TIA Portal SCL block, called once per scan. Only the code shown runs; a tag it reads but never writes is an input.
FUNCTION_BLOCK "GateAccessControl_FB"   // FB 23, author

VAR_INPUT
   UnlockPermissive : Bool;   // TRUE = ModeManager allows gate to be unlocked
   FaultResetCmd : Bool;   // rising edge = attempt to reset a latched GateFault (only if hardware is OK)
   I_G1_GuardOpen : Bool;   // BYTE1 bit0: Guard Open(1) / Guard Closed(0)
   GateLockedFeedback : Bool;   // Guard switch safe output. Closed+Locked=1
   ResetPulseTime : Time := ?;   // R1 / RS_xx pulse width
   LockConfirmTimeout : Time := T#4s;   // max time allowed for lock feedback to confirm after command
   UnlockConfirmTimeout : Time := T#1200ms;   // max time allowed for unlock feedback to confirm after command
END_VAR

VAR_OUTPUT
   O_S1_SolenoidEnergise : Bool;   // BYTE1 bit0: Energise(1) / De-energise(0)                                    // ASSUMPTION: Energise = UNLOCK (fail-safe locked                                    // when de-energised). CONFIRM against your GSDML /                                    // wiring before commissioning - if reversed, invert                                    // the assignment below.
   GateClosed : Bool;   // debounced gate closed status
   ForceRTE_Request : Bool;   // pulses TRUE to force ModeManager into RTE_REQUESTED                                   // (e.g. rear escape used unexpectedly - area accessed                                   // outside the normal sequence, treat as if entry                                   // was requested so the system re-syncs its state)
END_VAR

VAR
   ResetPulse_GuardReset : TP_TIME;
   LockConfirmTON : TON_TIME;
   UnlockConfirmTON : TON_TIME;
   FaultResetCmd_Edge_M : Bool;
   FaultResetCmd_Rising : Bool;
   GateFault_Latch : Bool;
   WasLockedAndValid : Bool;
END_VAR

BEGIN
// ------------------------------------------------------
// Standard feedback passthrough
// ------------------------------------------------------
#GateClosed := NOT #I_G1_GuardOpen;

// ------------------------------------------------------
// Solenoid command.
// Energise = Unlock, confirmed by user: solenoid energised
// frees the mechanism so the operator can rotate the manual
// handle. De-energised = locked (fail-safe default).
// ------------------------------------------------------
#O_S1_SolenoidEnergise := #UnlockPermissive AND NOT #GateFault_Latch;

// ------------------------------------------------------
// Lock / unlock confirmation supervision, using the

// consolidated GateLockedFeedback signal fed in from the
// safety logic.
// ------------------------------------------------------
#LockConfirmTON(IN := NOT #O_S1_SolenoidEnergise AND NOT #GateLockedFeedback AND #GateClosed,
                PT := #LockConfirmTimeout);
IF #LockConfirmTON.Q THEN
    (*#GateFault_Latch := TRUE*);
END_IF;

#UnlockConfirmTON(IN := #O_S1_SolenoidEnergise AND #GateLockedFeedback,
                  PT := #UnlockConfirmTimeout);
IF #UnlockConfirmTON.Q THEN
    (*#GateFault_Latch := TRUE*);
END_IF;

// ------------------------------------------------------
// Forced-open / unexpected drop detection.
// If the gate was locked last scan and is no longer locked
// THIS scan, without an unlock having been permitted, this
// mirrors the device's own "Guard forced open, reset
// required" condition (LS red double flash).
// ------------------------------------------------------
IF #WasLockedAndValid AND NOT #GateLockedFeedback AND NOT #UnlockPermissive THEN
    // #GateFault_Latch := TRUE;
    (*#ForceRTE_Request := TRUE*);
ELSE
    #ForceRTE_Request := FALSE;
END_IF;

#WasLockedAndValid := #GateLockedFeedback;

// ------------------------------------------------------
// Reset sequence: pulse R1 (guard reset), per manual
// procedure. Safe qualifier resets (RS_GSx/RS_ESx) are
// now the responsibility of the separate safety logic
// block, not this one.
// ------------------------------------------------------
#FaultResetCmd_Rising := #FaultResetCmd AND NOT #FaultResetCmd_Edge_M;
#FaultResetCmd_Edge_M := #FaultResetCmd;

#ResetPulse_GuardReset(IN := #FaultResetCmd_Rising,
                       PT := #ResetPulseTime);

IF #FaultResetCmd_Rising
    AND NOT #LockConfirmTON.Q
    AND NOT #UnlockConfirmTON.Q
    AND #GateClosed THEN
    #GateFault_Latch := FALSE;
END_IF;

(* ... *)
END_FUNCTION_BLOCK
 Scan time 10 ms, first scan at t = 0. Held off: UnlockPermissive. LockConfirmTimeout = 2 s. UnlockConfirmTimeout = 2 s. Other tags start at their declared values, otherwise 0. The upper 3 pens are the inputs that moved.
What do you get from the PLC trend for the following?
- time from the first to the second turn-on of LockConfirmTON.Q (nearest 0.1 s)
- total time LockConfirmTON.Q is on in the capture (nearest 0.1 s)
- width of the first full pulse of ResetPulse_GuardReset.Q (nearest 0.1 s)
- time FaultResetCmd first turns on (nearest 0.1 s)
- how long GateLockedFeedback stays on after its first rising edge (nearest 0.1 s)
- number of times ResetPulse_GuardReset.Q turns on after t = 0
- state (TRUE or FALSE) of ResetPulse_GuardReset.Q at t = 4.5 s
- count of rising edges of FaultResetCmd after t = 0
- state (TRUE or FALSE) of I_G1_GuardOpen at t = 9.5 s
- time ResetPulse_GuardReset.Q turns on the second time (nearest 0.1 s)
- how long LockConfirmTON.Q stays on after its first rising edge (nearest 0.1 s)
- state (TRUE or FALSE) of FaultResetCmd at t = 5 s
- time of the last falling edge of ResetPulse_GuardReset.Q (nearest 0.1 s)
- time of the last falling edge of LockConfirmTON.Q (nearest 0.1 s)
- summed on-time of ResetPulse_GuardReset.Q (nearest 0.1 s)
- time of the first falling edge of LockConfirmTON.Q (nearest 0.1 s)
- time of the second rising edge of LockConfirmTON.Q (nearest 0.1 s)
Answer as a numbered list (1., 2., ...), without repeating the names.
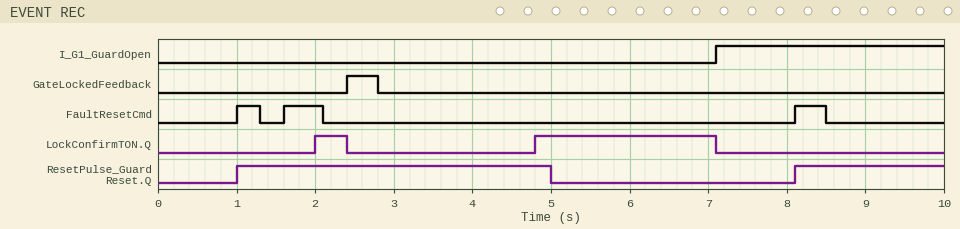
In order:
1. 2.8 s
2. 2.7 s
3. 4.0 s
4. 1.0 s
5. 0.4 s
6. 2
7. TRUE
8. 3
9. TRUE
10. 8.1 s
11. 0.4 s
12. FALSE
13. 5.0 s
14. 7.1 s
15. 5.9 s
16. 2.4 s
17. 4.8 s
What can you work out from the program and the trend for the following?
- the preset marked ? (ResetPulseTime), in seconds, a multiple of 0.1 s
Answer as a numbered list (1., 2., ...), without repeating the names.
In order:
1. 4.0 s
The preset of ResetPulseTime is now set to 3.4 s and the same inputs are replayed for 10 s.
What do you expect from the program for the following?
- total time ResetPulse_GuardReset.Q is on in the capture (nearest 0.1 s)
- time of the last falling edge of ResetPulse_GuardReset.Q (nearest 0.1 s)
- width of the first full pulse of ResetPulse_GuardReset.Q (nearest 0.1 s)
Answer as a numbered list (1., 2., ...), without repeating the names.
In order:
1. 5.3 s
2. 4.4 s
3. 3.4 s
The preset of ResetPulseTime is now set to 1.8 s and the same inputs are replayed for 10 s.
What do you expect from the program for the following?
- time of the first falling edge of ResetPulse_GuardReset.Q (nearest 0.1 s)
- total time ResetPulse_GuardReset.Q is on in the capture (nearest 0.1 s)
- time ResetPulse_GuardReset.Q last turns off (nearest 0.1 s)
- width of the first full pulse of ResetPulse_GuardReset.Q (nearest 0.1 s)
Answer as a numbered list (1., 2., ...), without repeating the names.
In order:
1. 2.8 s
2. 3.6 s
3. 9.9 s
4. 1.8 s
